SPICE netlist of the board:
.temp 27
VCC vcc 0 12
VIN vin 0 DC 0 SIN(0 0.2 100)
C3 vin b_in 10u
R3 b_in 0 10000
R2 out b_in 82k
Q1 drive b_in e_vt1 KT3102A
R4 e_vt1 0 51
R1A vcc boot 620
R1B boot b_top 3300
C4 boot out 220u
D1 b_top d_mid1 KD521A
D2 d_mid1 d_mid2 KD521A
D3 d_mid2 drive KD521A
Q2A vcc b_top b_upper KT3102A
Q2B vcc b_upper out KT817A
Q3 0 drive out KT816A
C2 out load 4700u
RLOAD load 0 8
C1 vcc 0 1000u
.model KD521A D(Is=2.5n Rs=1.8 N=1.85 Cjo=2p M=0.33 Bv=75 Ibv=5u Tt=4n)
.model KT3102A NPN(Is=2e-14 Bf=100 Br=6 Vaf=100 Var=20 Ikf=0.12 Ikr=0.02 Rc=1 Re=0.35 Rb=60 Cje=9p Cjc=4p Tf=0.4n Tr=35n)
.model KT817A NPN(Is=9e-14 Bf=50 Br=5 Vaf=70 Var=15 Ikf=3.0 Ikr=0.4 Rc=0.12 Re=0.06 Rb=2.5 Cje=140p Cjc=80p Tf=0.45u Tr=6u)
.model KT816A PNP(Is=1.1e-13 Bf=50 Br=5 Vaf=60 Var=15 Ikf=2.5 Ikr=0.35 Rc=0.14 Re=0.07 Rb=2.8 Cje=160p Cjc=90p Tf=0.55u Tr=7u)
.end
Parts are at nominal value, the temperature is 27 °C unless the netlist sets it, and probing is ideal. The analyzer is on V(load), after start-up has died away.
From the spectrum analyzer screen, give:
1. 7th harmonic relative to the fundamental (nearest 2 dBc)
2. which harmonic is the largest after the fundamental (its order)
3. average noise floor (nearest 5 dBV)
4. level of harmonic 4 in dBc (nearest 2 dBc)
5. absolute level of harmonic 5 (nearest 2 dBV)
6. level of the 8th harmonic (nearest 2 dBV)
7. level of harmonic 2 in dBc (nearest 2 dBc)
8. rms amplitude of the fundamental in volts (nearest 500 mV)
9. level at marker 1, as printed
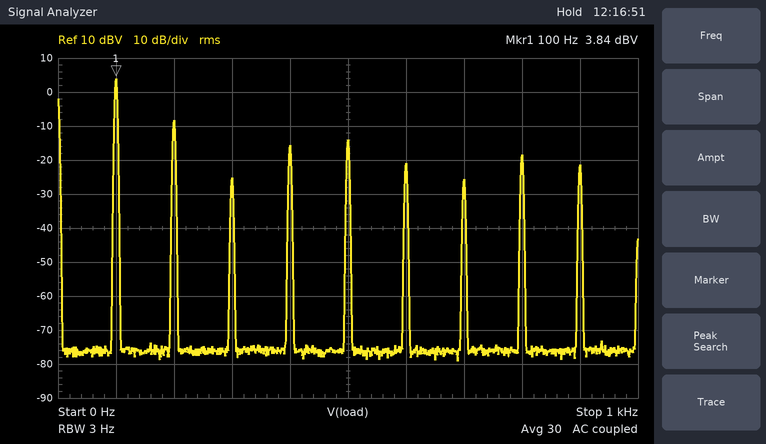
-30 dBc
2
-75 dBV
-20 dBc
-14 dBV
-18 dBV
-12 dBc
1.5 V
3.84 dBV
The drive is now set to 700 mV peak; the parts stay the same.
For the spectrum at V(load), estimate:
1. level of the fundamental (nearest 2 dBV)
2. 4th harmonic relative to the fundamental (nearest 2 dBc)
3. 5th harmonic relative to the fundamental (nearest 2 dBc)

8 dBV
-24 dBc
-22 dBc
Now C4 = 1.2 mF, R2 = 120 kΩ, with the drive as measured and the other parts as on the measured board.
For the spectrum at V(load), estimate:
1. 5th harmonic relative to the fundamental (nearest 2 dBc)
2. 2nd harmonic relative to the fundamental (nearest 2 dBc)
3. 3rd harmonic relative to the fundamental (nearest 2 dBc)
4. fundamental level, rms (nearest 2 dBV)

-42 dBc
-36 dBc
-20 dBc
0 dBV
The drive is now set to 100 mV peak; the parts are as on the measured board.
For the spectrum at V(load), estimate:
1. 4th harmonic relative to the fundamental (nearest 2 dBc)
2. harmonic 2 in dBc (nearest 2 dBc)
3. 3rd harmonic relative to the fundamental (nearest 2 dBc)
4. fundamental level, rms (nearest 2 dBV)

-12 dBc
-6 dBc
-8 dBc
0 dBV
